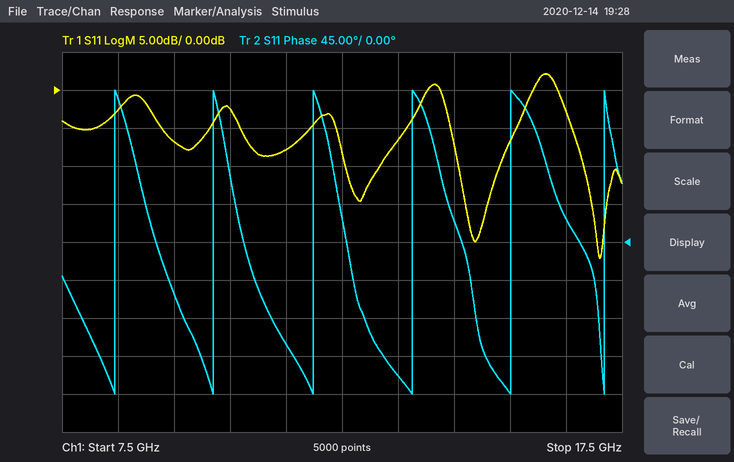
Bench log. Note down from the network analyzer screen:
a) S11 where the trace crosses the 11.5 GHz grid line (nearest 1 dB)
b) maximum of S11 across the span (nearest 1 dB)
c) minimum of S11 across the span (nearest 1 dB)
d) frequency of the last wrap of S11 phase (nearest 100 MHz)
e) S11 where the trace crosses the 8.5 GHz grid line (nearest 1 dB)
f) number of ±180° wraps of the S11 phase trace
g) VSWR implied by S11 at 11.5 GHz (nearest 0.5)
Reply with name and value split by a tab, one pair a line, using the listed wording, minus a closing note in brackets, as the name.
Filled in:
S11 where the trace crosses the 11.5 GHz grid line	-8 dB
maximum of S11 across the span	2 dB
minimum of S11 across the span	-22 dB
frequency of the last wrap of S11 phase	17.2 GHz
S11 where the trace crosses the 8.5 GHz grid line	-3 dB
number of ±180° wraps of the S11 phase trace	6
VSWR implied by S11 at 11.5 GHz	2.5
